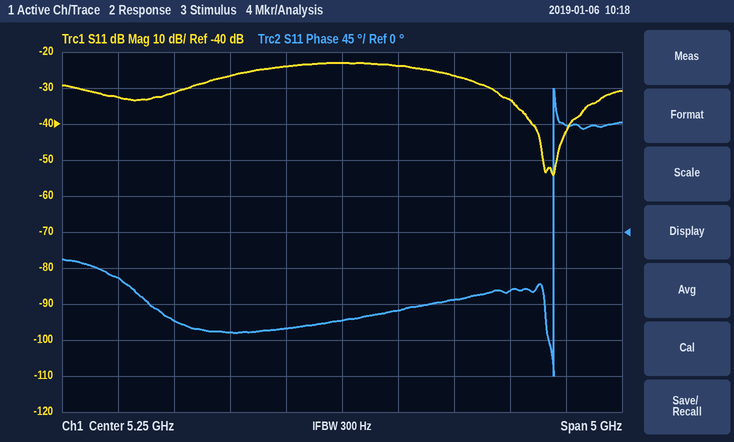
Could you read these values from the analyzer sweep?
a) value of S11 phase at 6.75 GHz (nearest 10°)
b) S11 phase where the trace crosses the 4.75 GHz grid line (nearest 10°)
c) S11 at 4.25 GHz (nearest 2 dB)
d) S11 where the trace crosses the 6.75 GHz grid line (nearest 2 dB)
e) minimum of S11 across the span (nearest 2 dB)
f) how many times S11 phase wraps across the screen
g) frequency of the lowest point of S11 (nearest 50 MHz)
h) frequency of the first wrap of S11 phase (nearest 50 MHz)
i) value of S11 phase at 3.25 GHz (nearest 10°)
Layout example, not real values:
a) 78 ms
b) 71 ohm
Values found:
a) -70°
b) -120°
c) -26 dB
d) -34 dB
e) -54 dB
f) 1
g) 7.15 GHz
h) 7.15 GHz
i) -60°
